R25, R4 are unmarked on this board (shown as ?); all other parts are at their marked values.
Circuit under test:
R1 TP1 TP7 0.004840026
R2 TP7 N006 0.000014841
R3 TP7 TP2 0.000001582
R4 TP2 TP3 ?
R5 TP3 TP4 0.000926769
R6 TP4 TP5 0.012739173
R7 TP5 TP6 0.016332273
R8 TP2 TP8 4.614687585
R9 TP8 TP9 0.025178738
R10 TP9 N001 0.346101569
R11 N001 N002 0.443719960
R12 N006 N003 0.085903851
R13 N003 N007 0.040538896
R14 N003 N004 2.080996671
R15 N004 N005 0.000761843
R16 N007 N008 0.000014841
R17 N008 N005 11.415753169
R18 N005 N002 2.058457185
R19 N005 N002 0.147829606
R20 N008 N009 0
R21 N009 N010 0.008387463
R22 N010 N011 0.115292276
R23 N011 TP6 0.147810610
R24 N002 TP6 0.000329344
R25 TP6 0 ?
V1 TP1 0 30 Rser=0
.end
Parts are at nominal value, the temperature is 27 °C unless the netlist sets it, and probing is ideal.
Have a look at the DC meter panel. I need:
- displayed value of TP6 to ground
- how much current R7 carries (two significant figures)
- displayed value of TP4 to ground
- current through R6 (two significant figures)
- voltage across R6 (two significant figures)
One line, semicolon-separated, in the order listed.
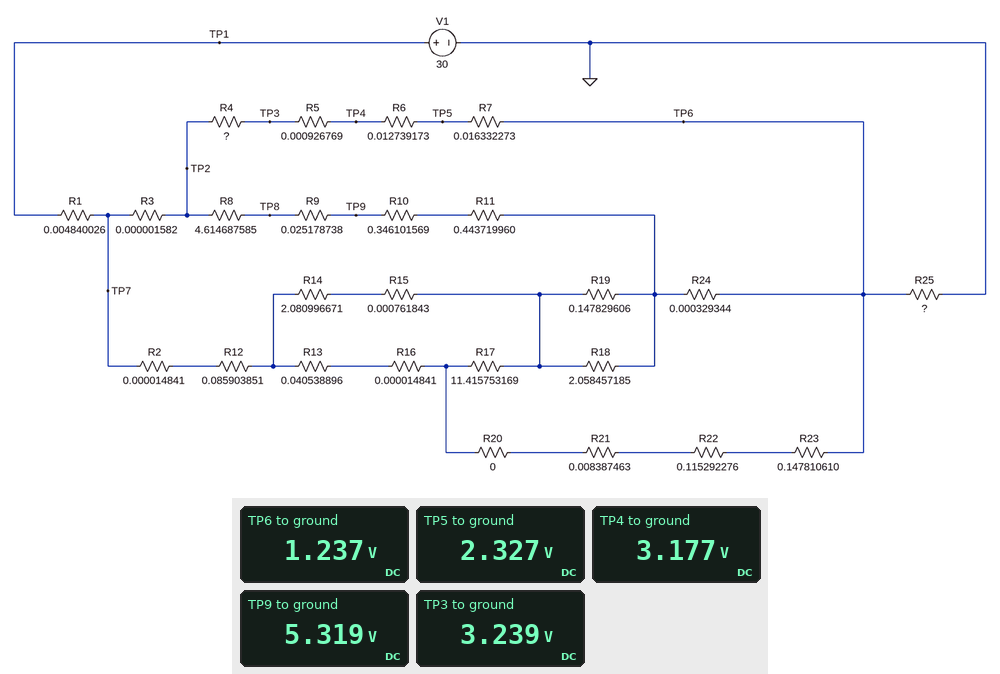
1.237 V; 67 A; 3.177 V; 67 A; 850 mV
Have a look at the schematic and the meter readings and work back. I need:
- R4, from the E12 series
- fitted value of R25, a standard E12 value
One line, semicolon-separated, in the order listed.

0.39 Ω; 8.2 mΩ
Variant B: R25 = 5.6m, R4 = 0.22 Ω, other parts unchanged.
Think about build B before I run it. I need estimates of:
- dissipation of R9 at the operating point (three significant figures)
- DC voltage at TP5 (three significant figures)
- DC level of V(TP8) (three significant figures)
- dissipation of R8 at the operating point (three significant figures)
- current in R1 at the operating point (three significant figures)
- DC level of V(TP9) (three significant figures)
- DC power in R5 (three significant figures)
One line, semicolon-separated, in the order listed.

667 mW; 2.92 V; 5.30 V; 122 W; 196 A; 5.17 V; 11.6 W
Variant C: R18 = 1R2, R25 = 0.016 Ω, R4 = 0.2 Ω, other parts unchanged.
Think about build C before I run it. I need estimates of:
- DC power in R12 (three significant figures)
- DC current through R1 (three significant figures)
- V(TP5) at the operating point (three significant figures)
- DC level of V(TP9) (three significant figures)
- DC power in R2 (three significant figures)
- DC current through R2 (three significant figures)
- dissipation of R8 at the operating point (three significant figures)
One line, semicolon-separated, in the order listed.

461 W; 191 A; 4.91 V; 6.85 V; 79.6 mW; 73.2 A; 106 W
